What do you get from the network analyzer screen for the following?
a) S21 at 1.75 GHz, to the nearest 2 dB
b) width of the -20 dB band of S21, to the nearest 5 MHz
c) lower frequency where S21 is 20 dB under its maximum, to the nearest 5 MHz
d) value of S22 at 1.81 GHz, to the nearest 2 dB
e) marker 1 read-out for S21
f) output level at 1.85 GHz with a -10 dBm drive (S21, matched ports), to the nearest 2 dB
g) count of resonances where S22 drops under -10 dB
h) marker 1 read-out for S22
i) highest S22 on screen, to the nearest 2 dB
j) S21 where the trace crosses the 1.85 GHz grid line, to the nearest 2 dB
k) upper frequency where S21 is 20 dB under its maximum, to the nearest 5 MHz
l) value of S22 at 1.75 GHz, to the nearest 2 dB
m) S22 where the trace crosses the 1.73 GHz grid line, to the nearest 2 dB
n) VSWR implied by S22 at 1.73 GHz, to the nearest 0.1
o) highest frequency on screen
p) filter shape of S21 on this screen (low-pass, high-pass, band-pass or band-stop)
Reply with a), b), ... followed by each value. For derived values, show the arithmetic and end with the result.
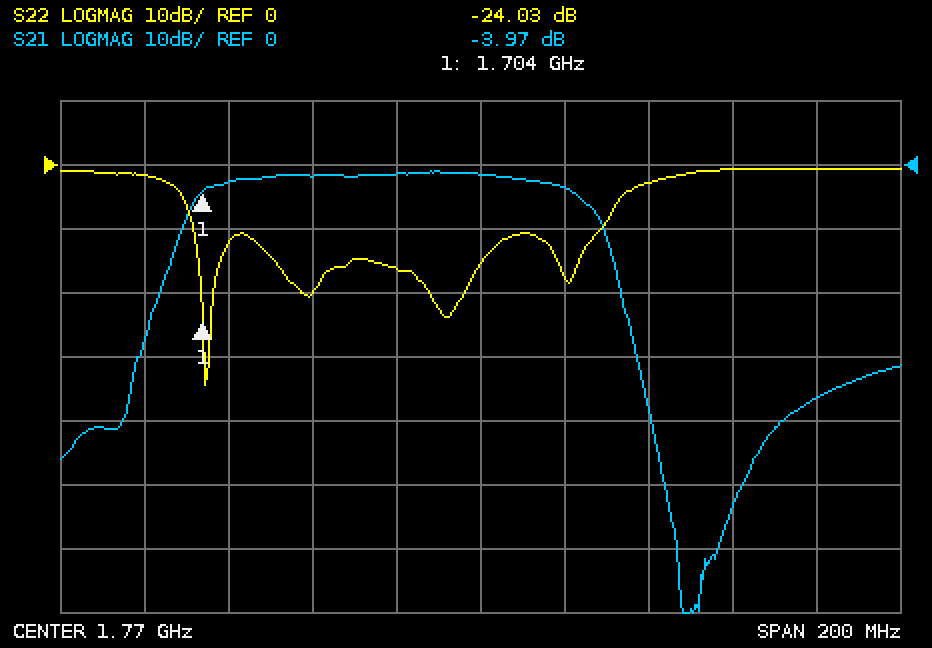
a) -2 dB
b) 1.805 GHz − 1.695 GHz = 110 MHz
c) 1.695 GHz
d) -2 dB
e) -3.97 dB
f) -10 dBm + (-36 dB) = -46 dBm
g) 4
h) -24.03 dB
i) 0 dB
j) -36 dB
k) 1.805 GHz
l) -16 dB
m) -20 dB
n) |Γ| = 10^(-20/20) = 0.1000; VSWR = (1 + 0.1000)/(1 − 0.1000) ≈ 1.2
o) 1.87 GHz
p) band-pass
